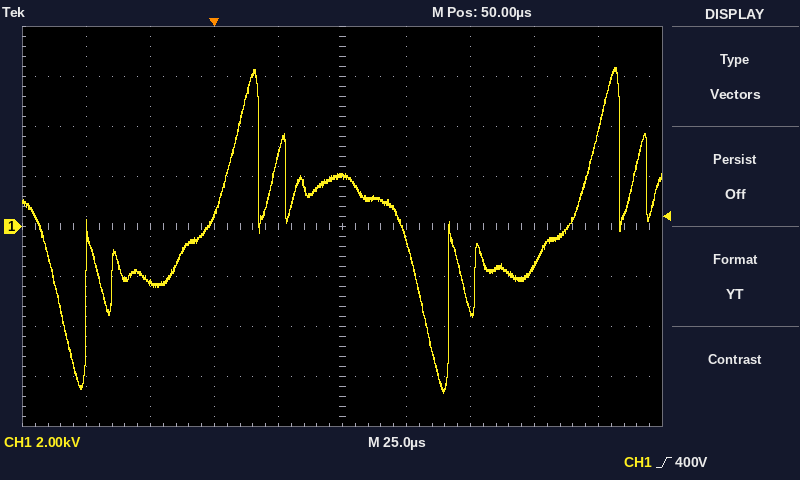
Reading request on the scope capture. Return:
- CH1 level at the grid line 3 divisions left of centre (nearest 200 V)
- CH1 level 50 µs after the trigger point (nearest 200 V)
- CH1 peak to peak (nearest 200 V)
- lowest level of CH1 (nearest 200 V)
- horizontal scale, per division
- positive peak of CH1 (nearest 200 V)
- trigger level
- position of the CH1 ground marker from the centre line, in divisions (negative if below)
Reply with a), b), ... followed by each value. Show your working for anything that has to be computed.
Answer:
a) -2.2 kV
b) 2.0 kV
c) 6.4 kV − (-6.6 kV) = 13.0 kV
d) -6.6 kV
e) 25 µs
f) 6.4 kV
g) 400 V
h) 0.0 div
